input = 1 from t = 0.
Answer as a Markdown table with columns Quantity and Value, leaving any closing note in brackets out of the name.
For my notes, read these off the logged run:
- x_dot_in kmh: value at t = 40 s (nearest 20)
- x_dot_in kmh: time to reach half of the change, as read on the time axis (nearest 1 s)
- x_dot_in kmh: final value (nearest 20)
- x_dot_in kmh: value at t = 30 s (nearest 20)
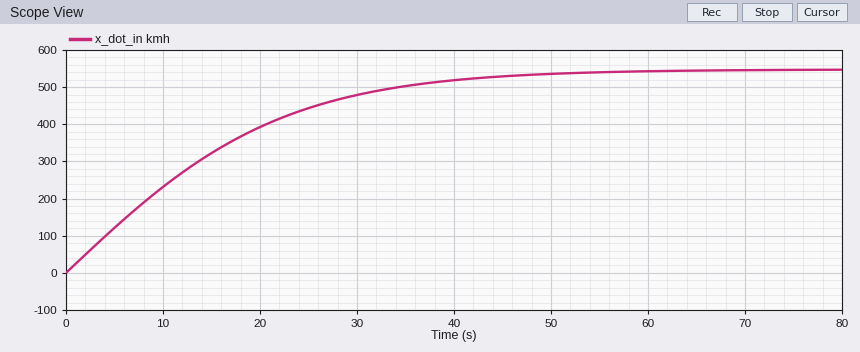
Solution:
| Quantity | Value |
|---|---|
| x_dot_in kmh: value at t = 40 s | 520 |
| x_dot_in kmh: time to reach half of the change, as read on the time axis | 12 s |
| x_dot_in kmh: final value | 540 |
| x_dot_in kmh: value at t = 30 s | 480 |
